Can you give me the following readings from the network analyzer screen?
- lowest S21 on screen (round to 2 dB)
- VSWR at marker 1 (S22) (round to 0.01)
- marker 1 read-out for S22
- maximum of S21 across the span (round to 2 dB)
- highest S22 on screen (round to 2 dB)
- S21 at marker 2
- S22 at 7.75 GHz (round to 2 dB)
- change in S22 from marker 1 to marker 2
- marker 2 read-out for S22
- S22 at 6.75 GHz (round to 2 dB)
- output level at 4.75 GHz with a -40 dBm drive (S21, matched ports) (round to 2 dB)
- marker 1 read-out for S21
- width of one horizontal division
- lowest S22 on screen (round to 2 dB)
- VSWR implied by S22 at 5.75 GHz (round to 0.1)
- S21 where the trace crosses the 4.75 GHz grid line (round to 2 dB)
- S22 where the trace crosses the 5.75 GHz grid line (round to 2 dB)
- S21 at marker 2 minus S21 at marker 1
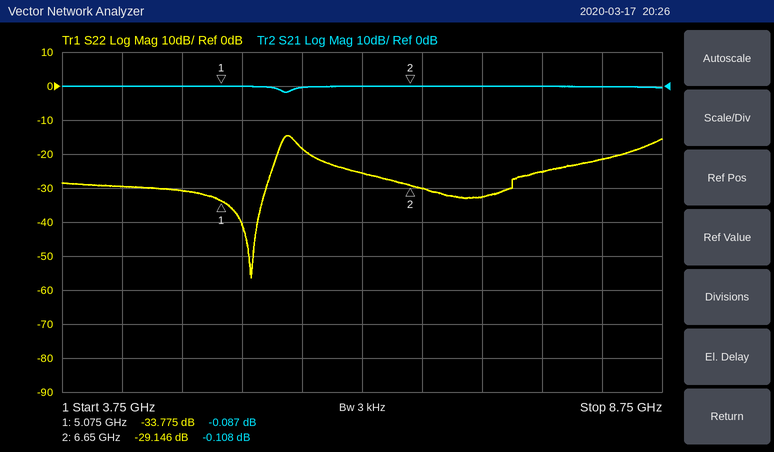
-2 dB
1.04
-33.775 dB
0 dB
-14 dB
-0.108 dB
-26 dB
4.629 dB
-29.146 dB
-30 dB
-40 dBm
-0.087 dB
500 MHz
-56 dB
1.3
0 dB
-18 dB
-0.021 dB
